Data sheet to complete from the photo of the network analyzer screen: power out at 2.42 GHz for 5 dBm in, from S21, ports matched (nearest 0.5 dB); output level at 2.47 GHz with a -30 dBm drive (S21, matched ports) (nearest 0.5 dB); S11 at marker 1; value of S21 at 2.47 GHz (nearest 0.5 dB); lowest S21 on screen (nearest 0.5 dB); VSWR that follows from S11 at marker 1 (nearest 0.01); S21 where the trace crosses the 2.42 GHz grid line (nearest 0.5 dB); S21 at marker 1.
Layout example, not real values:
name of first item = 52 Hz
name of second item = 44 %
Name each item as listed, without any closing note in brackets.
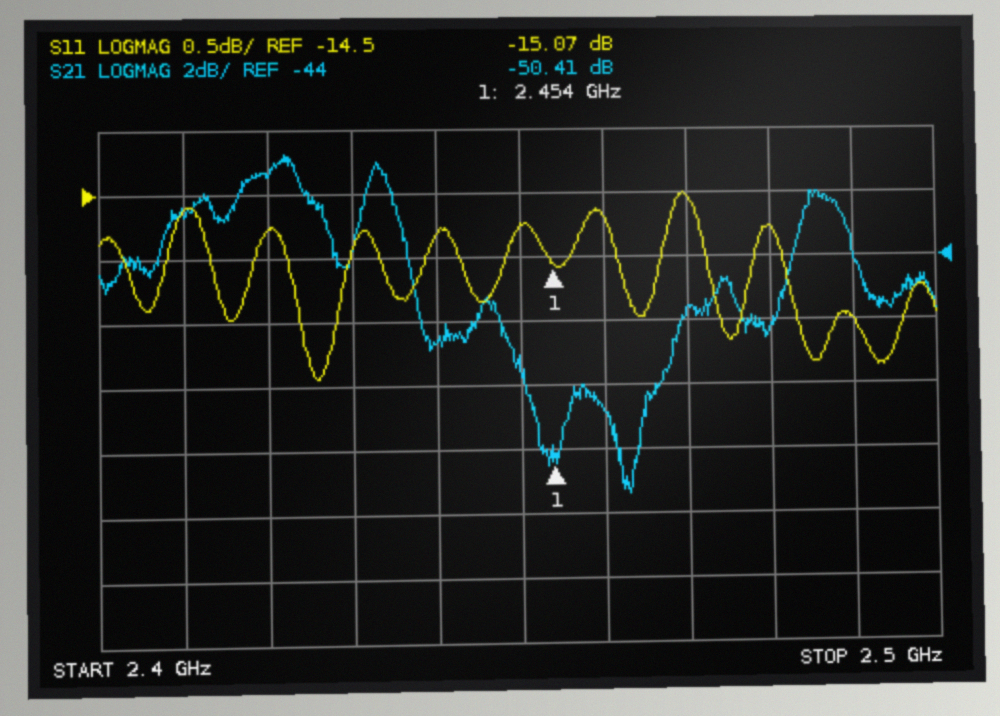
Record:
power out at 2.42 GHz for 5 dBm in, from S21, ports matched = -36.5 dBm
output level at 2.47 GHz with a -30 dBm drive (S21, matched ports) = -75.5 dBm
S11 at marker 1 = -15.07 dB
value of S21 at 2.47 GHz = -45.5 dB
lowest S21 on screen = -51.5 dB
VSWR that follows from S11 at marker 1 = 1.43
S21 where the trace crosses the 2.42 GHz grid line = -41.5 dB
S21 at marker 1 = -50.41 dB
